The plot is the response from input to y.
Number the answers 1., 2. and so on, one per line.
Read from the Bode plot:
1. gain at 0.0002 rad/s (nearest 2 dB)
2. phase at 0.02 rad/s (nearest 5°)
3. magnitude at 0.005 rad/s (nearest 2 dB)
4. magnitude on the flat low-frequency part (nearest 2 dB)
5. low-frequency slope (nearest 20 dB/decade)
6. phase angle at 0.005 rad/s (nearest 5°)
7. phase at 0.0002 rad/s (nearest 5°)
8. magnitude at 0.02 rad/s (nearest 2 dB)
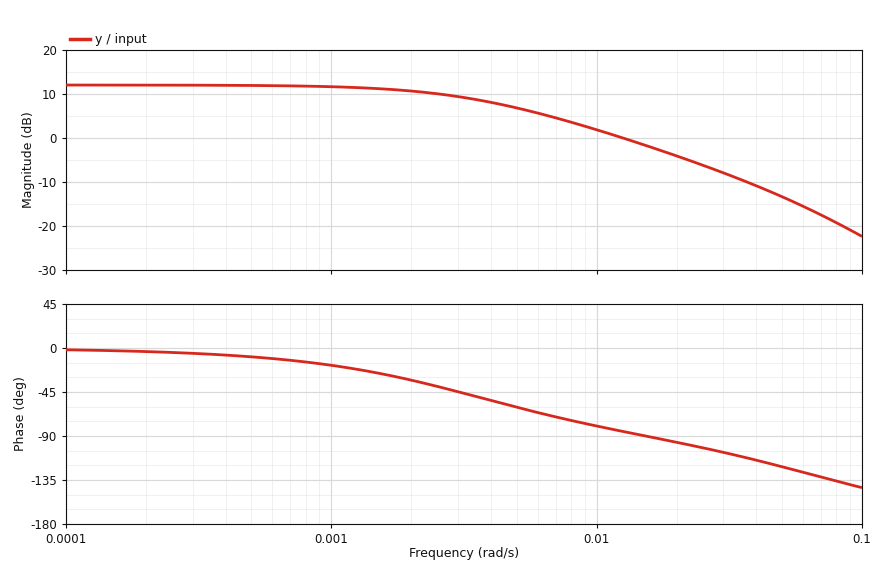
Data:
1. 12 dB
2. -95°
3. 6 dB
4. 12 dB
5. 0 dB/decade
6. -60°
7. -5°
8. -4 dB
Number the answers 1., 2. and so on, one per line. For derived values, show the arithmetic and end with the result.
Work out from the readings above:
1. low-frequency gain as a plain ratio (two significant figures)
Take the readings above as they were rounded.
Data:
1. 10^(12 / 20) = 4.0
